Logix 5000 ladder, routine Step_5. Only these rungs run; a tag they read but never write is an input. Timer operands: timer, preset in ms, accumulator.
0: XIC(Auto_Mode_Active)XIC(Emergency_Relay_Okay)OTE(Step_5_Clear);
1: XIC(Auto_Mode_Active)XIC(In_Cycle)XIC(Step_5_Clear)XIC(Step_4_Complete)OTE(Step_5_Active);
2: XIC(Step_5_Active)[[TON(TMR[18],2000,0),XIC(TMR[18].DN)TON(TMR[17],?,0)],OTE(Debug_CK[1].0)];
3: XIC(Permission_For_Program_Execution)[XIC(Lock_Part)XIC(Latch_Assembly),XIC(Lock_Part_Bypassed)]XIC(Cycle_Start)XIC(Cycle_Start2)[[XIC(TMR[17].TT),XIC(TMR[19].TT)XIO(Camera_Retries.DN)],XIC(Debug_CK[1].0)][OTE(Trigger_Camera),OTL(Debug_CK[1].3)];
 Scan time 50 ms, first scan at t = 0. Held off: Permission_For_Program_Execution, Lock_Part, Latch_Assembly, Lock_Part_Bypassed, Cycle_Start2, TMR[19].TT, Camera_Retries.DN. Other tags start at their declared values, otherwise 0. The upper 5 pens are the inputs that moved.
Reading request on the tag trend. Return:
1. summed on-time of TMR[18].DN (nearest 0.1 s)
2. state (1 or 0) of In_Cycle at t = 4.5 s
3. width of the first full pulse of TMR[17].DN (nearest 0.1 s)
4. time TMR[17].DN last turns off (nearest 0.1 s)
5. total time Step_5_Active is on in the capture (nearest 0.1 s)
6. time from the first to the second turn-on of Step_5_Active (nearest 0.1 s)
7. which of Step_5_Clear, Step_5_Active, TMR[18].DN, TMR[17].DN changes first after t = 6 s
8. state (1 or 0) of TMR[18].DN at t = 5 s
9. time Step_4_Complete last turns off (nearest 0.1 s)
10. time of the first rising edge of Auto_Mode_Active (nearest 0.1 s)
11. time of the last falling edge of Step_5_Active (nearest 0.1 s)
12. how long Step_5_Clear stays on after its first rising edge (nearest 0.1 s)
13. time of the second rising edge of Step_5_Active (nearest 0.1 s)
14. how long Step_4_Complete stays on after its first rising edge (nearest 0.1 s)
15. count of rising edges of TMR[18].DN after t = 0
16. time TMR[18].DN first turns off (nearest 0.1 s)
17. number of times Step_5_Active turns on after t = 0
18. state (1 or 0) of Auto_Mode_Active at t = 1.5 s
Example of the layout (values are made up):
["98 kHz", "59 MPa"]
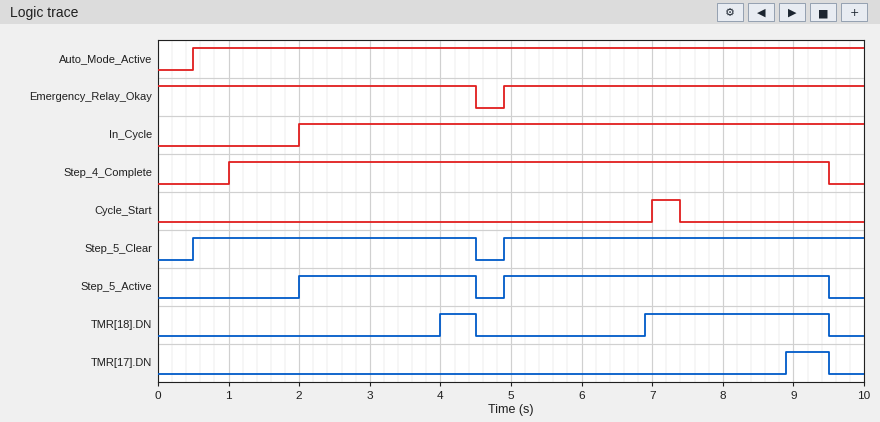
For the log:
["3.1 s", "1", "0.6 s", "9.5 s", "7.1 s", "2.9 s", "TMR[18].DN", "0", "9.5 s", "0.5 s", "9.5 s", "4.0 s", "4.9 s", "8.5 s", "2", "4.5 s", "2", "1"]
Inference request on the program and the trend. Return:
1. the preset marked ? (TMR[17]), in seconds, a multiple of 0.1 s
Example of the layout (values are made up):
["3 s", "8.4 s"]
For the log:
["2.0 s"]
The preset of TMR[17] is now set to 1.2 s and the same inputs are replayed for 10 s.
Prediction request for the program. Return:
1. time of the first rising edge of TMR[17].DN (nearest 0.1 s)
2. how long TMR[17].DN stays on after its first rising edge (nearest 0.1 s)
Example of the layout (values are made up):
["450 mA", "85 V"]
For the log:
["8.1 s", "1.4 s"]
